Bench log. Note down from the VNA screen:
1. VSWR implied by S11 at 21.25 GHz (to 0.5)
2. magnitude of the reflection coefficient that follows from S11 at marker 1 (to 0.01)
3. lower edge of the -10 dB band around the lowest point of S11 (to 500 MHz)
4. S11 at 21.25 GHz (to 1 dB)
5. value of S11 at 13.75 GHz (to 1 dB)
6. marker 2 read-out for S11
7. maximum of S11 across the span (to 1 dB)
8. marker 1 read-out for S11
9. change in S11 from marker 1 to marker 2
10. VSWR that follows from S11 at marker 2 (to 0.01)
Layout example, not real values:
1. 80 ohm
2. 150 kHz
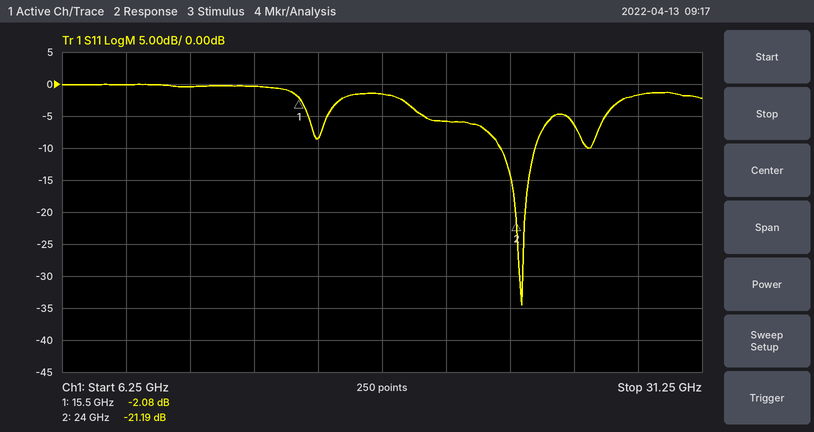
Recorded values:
1. 3.0
2. 0.79
3. 23.5 GHz
4. -6 dB
5. 0 dB
6. -21.19 dB
7. 0 dB
8. -2.08 dB
9. -19.11 dB
10. 1.19
